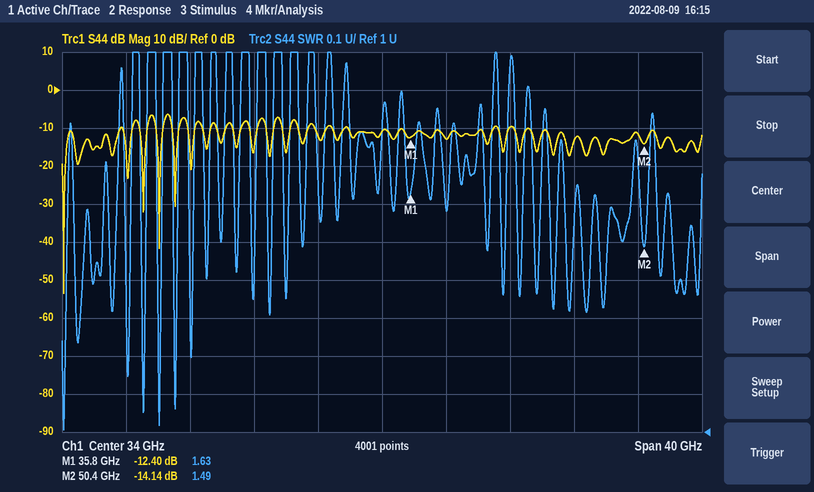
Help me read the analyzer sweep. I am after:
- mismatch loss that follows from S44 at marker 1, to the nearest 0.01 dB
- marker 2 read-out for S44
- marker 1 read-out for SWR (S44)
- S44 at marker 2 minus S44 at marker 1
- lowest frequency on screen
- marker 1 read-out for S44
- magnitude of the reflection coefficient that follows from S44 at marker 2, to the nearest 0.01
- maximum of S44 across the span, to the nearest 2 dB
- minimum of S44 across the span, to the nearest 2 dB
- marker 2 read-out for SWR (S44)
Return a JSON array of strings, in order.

["0.26 dB", "-14.14 dB", "1.63", "-1.74 dB", "14 GHz", "-12.40 dB", "0.20", "-6 dB", "-54 dB", "1.49"]
